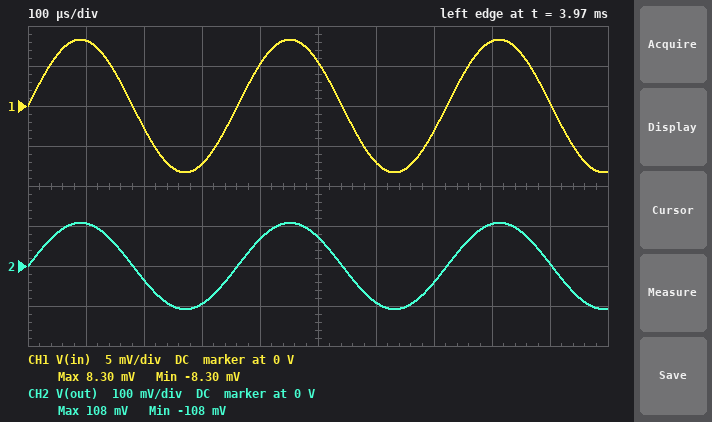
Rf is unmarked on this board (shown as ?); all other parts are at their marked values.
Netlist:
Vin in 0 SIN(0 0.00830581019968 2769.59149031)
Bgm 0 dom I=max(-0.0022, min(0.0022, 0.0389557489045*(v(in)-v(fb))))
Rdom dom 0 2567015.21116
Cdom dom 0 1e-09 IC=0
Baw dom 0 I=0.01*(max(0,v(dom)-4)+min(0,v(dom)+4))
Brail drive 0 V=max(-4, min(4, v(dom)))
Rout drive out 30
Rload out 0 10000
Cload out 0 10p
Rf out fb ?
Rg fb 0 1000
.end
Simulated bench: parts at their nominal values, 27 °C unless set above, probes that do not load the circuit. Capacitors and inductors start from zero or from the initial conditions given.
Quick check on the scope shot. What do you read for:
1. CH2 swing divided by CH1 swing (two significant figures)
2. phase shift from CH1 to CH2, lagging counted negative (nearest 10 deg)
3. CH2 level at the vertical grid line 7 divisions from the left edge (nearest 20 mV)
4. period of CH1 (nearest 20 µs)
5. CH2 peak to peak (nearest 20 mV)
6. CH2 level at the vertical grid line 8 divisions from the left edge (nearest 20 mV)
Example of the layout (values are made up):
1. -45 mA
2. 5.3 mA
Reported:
1. 13
2. 0 deg
3. -40 mV
4. 360 µs
5. 220 mV
6. 100 mV
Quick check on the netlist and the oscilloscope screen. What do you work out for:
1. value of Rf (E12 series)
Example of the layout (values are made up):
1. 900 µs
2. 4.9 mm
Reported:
1. 12 kΩ
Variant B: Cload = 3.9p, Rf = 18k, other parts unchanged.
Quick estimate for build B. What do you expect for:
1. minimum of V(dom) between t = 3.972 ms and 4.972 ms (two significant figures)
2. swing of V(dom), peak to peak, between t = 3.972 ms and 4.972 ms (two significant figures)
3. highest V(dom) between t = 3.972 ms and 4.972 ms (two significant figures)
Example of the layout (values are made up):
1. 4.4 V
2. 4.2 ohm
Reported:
1. -160 mV
2. 320 mV
3. 160 mV
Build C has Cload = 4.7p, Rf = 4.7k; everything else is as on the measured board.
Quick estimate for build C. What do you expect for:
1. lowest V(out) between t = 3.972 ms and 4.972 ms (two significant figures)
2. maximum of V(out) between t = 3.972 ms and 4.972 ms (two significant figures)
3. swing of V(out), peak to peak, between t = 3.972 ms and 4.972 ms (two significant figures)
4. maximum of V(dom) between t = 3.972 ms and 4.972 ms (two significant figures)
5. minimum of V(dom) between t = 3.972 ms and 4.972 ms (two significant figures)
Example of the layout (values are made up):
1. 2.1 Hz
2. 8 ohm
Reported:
1. -47 mV
2. 47 mV
3. 95 mV
4. 48 mV
5. -48 mV
